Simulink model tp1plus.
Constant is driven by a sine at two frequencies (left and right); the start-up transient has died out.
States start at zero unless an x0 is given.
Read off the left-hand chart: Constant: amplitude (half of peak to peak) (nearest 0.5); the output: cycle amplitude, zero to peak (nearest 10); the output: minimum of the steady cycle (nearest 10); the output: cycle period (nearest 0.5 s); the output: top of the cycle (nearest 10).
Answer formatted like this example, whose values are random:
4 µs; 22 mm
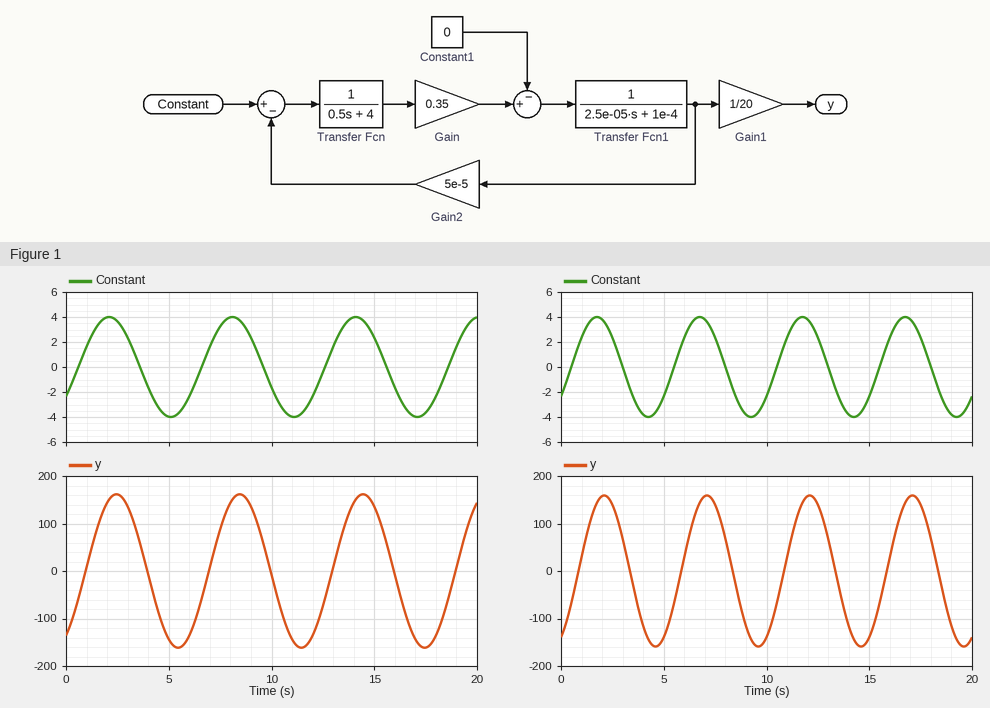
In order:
4.0; 160; -160; 6.0 s; 160
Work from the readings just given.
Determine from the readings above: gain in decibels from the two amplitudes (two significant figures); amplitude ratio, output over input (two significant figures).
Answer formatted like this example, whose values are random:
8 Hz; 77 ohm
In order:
32 dB; 40
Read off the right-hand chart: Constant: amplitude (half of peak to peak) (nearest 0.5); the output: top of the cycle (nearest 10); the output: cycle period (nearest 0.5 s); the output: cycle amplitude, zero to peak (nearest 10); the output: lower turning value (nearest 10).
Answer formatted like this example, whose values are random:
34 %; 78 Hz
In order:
4.0; 160; 5.0 s; 160; -160
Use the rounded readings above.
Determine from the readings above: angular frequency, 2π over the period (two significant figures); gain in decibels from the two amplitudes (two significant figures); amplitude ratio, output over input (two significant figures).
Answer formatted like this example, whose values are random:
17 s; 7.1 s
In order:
1.3 rad/s; 32 dB; 40
